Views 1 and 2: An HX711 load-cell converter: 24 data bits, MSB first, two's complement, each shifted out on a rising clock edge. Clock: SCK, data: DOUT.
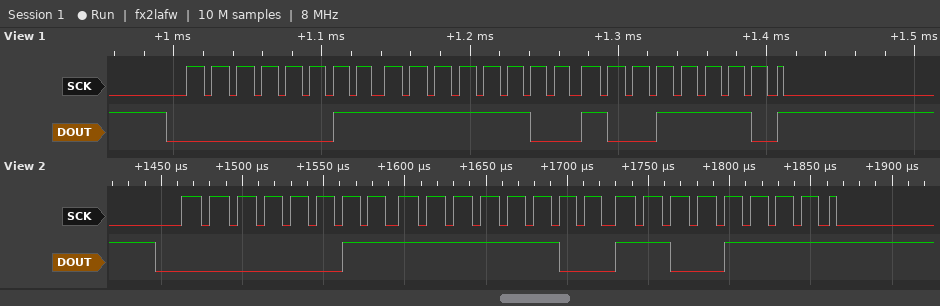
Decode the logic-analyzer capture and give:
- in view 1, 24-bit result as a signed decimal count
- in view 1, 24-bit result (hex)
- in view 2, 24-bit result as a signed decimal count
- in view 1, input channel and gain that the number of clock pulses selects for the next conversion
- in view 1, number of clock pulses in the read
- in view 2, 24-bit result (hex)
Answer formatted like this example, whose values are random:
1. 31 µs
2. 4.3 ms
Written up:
1. 261278
2. 0x03FC9E
3. 261327
4. channel A, gain 128
5. 25
6. 0x03FCCF
